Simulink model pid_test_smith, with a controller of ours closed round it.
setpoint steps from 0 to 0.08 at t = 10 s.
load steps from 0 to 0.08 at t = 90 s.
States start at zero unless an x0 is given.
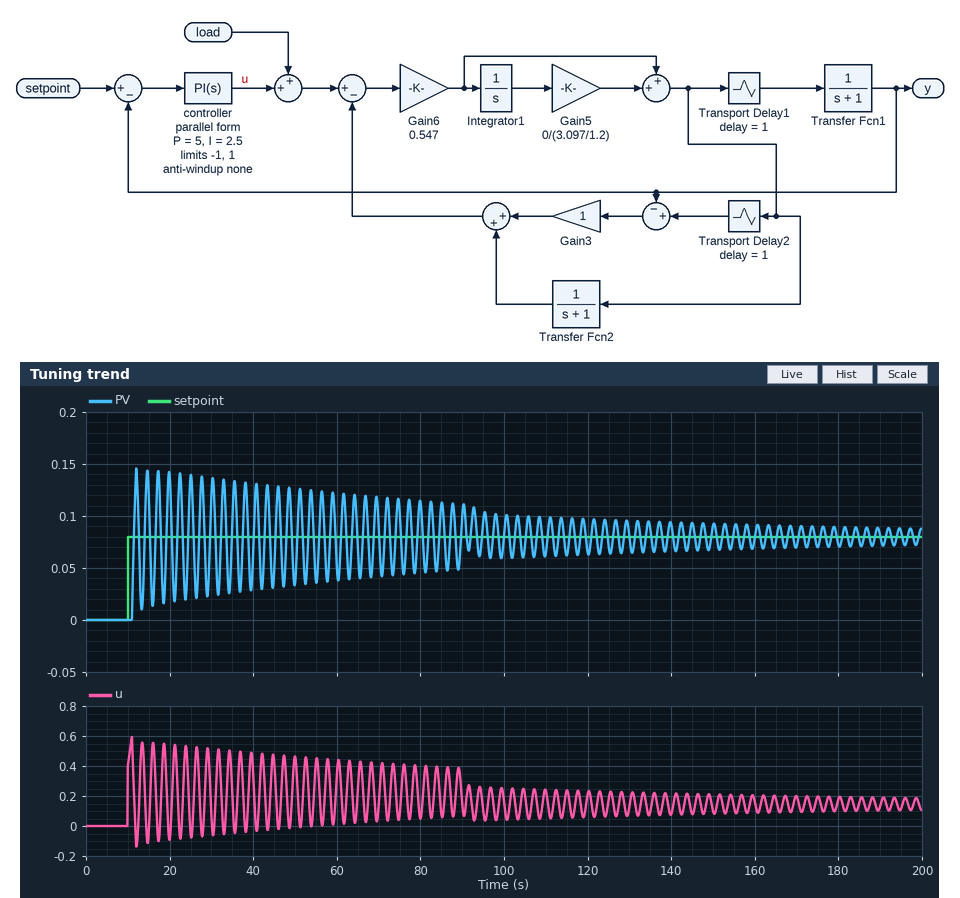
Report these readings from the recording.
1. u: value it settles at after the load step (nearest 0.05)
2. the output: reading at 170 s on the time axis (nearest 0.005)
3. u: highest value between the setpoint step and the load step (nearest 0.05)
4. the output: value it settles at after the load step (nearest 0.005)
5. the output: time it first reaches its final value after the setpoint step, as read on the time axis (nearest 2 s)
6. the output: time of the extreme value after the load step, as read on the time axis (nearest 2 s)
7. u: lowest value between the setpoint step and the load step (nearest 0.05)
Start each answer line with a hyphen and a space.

- 0.15
- 0.070
- 0.60
- 0.080
- 12 s
- 90 s
- -0.15
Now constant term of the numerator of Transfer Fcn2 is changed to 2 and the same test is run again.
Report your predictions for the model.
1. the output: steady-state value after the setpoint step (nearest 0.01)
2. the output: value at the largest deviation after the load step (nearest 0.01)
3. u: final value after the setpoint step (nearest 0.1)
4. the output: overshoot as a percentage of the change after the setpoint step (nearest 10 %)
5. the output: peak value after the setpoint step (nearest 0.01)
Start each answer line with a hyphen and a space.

- 0.08
- 0.10
- 0.3
- 50 %
- 0.12
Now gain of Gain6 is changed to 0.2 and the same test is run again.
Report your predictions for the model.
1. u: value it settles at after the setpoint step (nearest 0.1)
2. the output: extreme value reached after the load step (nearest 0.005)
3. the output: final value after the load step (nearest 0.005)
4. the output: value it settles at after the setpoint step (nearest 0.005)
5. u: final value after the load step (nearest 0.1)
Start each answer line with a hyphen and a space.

- 0.5
- 0.090
- 0.080
- 0.080
- 0.4
